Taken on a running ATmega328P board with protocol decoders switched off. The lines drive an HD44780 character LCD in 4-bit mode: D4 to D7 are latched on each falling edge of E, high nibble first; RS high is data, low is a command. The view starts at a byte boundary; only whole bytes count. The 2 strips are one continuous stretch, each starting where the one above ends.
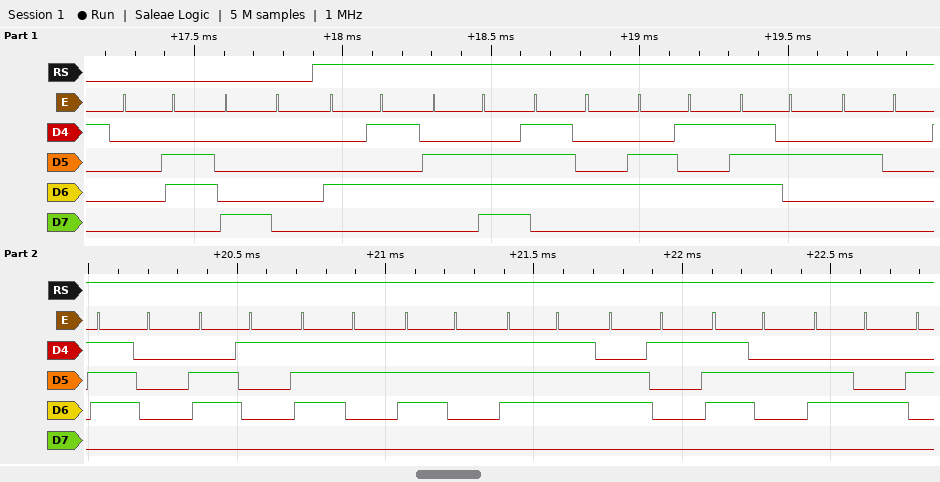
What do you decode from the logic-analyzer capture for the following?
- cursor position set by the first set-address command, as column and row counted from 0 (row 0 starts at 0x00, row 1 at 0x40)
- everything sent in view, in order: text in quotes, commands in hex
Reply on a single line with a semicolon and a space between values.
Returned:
column 0, row 0; 0x06 0x80 "Enter passward"
